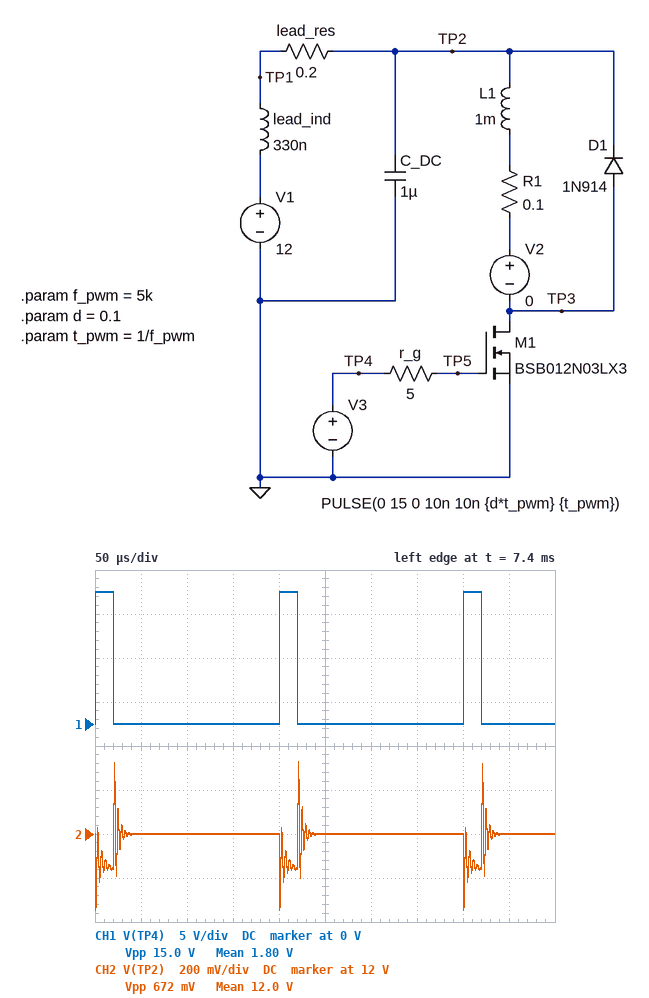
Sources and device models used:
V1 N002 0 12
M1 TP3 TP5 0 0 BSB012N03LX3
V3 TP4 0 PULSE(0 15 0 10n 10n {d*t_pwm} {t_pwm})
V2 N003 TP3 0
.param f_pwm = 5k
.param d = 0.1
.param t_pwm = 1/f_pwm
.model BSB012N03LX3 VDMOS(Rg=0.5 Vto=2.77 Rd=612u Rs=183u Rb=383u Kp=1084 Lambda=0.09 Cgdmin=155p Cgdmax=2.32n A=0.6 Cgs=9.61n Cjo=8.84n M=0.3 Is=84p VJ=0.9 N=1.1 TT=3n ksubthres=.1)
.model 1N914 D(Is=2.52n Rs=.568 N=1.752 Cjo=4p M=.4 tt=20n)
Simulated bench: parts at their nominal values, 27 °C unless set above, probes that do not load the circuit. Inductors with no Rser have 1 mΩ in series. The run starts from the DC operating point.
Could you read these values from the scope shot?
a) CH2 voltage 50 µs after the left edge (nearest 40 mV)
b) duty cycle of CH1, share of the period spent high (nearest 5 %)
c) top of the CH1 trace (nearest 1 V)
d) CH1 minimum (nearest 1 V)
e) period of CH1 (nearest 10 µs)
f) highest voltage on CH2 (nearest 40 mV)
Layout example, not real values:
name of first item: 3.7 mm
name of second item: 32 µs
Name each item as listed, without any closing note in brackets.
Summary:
CH2 voltage 50 µs after the left edge: 12.00 V
duty cycle of CH1, share of the period spent high: 10 %
top of the CH1 trace: 15 V
CH1 minimum: 0 V
period of CH1: 200 µs
highest voltage on CH2: 12.32 V
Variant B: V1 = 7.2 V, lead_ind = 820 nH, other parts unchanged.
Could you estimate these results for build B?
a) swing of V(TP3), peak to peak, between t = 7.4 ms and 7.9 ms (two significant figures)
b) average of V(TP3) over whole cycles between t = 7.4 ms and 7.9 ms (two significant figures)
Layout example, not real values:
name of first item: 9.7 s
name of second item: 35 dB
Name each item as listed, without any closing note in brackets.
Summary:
swing of V(TP3), peak to peak, between t = 7.4 ms and 7.9 ms: 8.2 V
average of V(TP3) over whole cycles between t = 7.4 ms and 7.9 ms: 7.2 V
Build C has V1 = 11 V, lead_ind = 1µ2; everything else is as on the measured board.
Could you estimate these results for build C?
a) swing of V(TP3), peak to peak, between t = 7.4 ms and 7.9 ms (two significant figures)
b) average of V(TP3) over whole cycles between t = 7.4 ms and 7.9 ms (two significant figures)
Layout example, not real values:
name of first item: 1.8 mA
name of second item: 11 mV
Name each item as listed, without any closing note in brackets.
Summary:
swing of V(TP3), peak to peak, between t = 7.4 ms and 7.9 ms: 13 V
average of V(TP3) over whole cycles between t = 7.4 ms and 7.9 ms: 11 V
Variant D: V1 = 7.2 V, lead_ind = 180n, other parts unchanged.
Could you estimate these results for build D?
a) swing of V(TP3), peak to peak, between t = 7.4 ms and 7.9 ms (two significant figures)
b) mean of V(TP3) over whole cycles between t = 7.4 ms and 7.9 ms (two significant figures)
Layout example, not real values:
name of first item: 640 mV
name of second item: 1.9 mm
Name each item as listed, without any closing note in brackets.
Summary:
swing of V(TP3), peak to peak, between t = 7.4 ms and 7.9 ms: 8.1 V
mean of V(TP3) over whole cycles between t = 7.4 ms and 7.9 ms: 7.2 V
